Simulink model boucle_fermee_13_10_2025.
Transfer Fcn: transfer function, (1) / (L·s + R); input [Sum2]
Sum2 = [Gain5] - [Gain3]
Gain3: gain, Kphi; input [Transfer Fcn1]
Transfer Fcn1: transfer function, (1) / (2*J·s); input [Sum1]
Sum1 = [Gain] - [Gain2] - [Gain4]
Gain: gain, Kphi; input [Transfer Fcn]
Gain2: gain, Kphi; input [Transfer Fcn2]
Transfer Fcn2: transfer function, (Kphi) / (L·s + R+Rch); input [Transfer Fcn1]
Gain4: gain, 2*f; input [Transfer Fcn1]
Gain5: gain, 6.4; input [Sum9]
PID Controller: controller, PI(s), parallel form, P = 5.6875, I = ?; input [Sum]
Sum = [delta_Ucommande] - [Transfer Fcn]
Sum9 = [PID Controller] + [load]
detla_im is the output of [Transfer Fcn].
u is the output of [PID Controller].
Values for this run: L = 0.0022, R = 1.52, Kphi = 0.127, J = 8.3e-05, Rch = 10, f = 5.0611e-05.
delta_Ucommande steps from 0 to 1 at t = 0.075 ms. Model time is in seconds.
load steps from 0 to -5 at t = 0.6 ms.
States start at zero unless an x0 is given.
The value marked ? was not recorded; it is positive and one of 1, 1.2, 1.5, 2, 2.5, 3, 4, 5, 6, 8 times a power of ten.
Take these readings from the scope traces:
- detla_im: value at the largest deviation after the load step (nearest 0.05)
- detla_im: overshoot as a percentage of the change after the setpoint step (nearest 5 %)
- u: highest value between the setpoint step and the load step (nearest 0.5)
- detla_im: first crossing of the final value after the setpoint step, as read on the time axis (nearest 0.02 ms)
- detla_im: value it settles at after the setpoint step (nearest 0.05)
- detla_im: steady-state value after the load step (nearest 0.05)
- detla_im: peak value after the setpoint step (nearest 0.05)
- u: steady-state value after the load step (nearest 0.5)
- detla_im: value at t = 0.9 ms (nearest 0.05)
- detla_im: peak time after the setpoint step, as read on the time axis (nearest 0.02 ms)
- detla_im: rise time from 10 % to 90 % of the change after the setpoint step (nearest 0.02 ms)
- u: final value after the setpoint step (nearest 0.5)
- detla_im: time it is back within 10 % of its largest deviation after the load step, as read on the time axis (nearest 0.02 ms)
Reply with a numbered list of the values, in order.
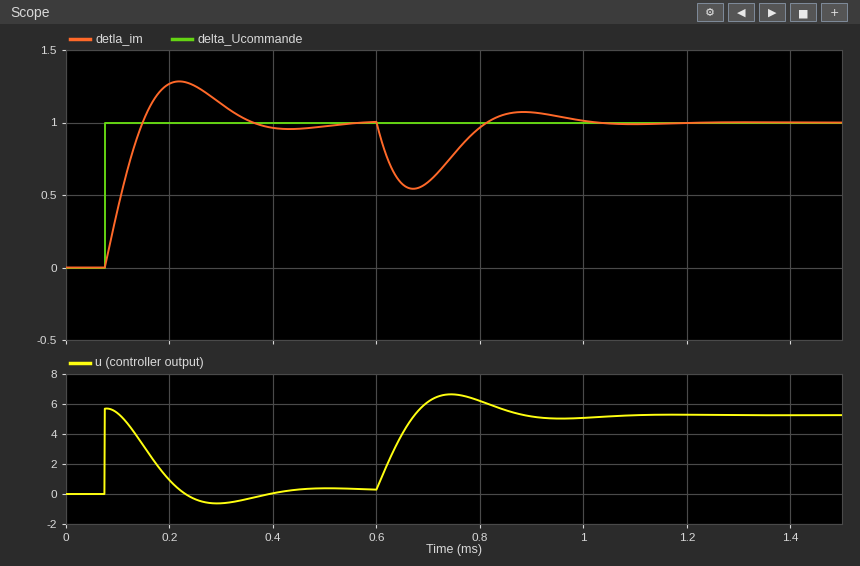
1. 0.55
2. 30 %
3. 5.5
4. 0.14 ms
5. 1.00
6. 1.00
7. 1.30
8. 5.5
9. 1.05
10. 0.22 ms
11. 0.06 ms
12. 0.5
13. 0.94 ms
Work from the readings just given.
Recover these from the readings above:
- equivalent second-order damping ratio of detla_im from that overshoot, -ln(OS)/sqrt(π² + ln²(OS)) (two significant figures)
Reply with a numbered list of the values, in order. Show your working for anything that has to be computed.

1. ln(0.3) = -1.204; 1.204 / sqrt(9.870 + 1.450) = 0.36
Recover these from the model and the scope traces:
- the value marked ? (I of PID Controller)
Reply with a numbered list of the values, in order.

1. 100000
